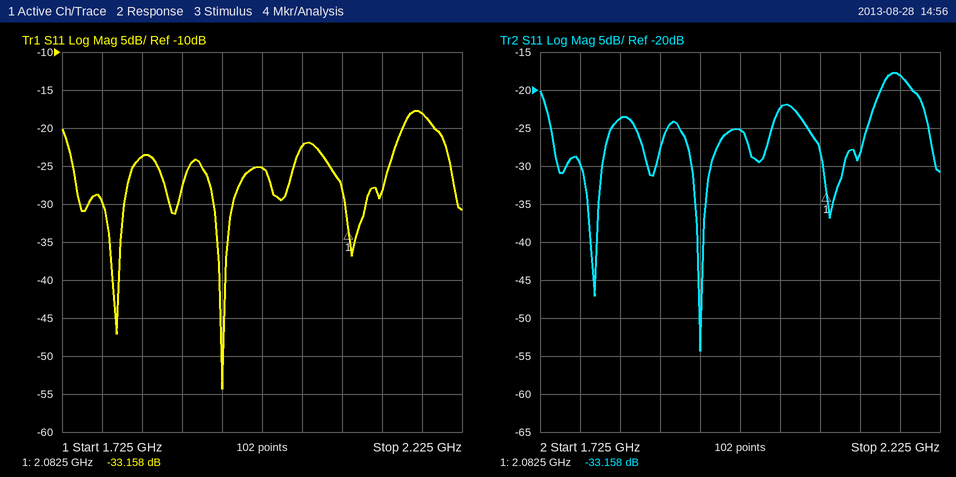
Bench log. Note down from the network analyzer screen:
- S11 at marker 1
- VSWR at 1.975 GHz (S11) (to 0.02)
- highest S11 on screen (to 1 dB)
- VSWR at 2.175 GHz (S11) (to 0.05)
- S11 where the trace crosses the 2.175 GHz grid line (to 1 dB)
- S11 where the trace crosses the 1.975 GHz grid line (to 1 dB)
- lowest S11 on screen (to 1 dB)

-33.158 dB
1.12
-18 dB
1.30
-18 dB
-25 dB
-54 dB
